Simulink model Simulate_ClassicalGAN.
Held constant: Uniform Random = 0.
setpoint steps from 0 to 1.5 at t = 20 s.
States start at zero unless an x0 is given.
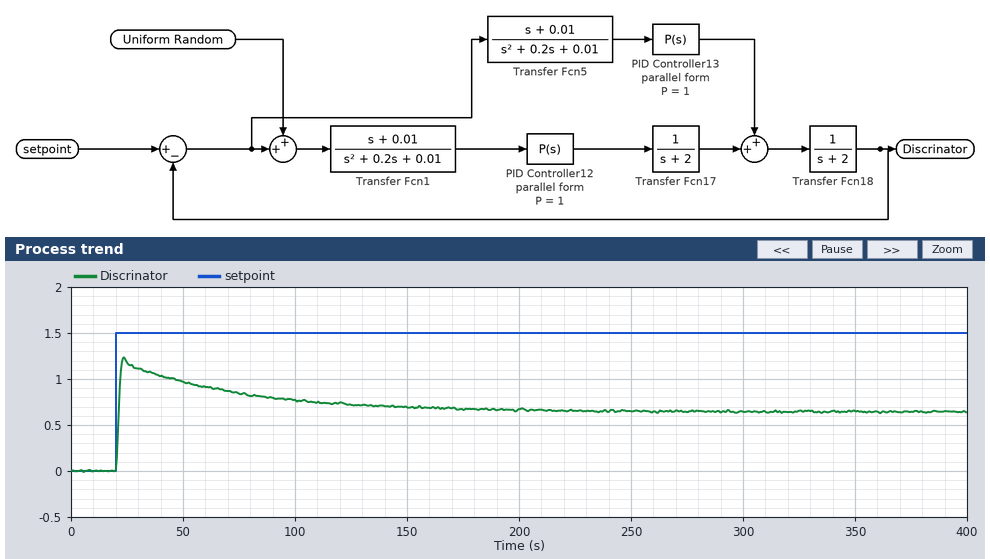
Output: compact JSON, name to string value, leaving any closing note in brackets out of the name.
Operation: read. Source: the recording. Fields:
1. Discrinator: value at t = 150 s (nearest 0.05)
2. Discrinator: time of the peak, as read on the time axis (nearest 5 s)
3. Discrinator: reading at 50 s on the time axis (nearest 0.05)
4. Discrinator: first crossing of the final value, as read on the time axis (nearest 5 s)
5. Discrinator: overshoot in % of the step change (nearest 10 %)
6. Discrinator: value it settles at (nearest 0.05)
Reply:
{"Discrinator: value at t = 150 s": "0.70", "Discrinator: time of the peak, as read on the time axis": "25 s", "Discrinator: reading at 50 s on the time axis": "0.95", "Discrinator: first crossing of the final value, as read on the time axis": "20 s", "Discrinator: overshoot in % of the step change": "90 %", "Discrinator: value it settles at": "0.65"}
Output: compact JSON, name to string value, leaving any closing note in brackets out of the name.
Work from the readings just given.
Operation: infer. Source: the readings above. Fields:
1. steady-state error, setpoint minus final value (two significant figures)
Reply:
{"steady-state error, setpoint minus final value": "0.85"}
